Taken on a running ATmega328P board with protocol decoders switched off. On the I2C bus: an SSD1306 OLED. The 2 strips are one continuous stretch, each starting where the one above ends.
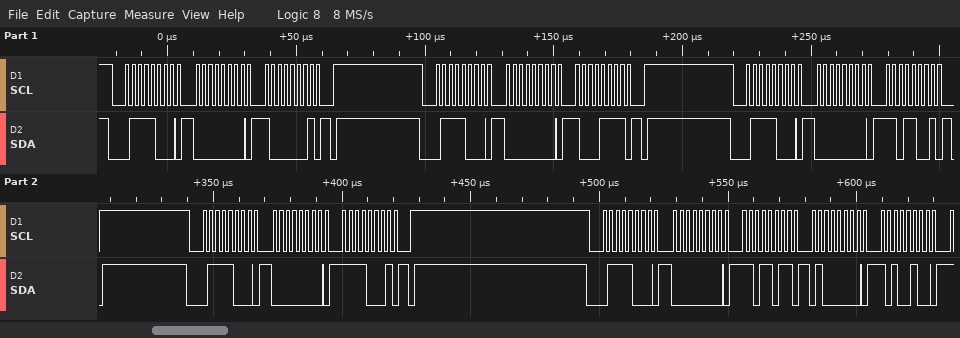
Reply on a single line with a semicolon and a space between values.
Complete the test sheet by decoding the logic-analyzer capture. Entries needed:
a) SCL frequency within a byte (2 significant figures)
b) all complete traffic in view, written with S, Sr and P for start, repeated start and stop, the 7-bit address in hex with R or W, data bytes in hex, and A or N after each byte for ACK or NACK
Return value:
400 kHz; S 3CW A 00 A 81 A P S 3CW A 00 A 8F A P S 3CW A 00 A D9 A P S 3CW A 00 A F1 A P S 3CW A 00 A DB A 40 A A4 A
